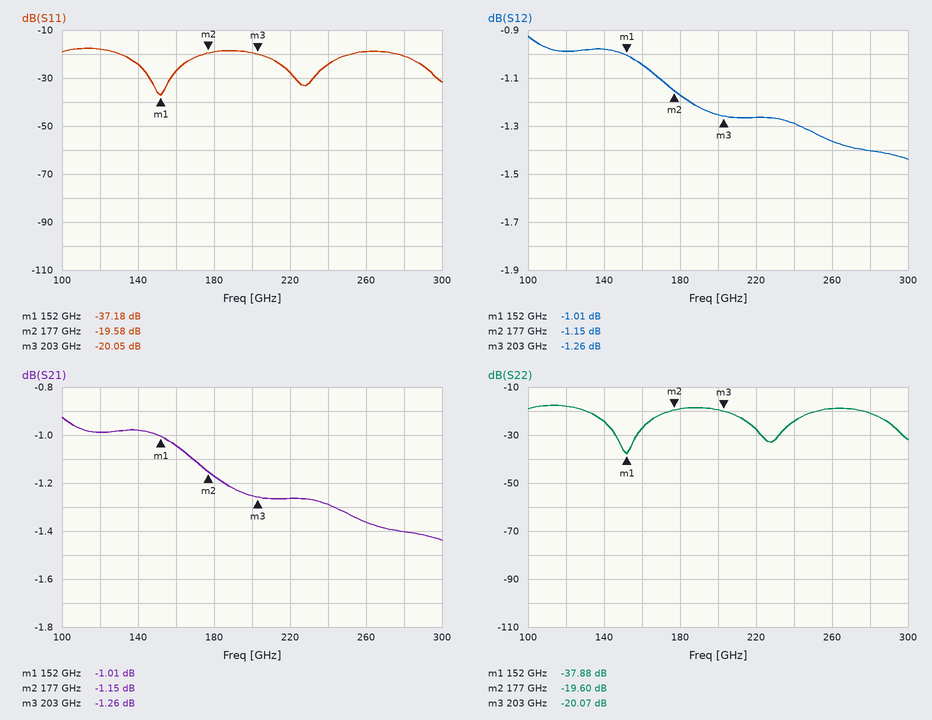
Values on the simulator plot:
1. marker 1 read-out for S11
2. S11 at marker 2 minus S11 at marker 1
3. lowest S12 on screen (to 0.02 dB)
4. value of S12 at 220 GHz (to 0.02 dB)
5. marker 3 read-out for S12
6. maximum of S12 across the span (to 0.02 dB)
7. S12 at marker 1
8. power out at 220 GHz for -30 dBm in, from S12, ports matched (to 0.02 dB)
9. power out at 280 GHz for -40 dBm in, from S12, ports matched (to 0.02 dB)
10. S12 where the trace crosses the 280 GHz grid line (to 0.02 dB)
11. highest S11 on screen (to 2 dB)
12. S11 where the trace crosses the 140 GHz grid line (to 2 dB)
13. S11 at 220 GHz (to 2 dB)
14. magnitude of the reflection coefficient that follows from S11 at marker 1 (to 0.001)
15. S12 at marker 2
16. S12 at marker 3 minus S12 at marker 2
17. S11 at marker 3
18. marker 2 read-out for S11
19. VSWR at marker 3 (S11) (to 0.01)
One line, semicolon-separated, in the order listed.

-37.18 dB; 17.60 dB; -1.44 dB; -1.26 dB; -1.26 dB; -0.92 dB; -1.01 dB; -31.26 dBm; -41.40 dBm; -1.40 dB; -18 dB; -24 dB; -28 dB; 0.014; -1.15 dB; -0.11 dB; -20.05 dB; -19.58 dB; 1.22
